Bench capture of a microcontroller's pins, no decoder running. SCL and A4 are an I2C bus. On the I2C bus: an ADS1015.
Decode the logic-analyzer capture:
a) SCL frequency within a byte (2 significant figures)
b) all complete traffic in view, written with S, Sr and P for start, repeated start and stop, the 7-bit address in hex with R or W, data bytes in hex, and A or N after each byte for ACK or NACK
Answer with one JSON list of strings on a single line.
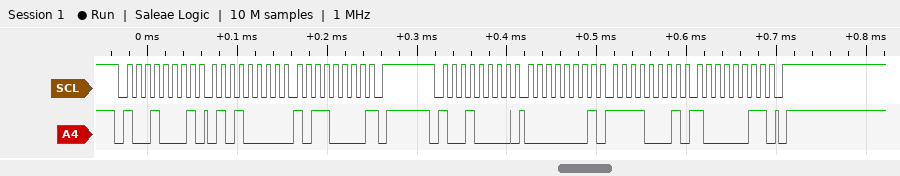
["100 kHz", "S 48R A 50 A B0 N P S 48W A 01 A F1 A 83 A P"]
